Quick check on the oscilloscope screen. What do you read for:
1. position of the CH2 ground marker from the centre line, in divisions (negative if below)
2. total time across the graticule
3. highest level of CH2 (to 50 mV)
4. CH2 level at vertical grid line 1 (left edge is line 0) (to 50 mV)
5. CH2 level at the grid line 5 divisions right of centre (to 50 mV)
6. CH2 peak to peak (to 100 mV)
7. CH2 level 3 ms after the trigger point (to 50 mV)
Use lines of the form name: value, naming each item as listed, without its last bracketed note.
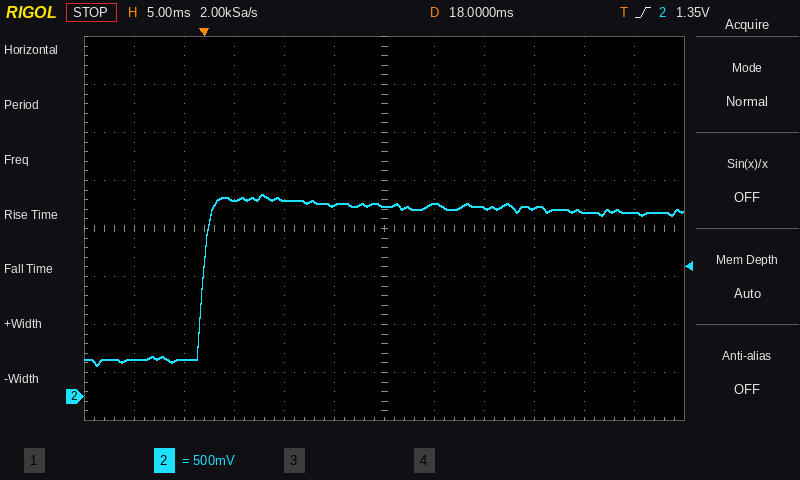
position of the CH2 ground marker from the centre line, in divisions: -3.5 div
total time across the graticule: 60 ms
highest level of CH2: 2.10 V
CH2 level at vertical grid line 1 (left edge is line 0): 400 mV
CH2 level at the grid line 5 divisions right of centre: 1.90 V
CH2 peak to peak: 1.80 V
CH2 level 3 ms after the trigger point: 2.05 V
